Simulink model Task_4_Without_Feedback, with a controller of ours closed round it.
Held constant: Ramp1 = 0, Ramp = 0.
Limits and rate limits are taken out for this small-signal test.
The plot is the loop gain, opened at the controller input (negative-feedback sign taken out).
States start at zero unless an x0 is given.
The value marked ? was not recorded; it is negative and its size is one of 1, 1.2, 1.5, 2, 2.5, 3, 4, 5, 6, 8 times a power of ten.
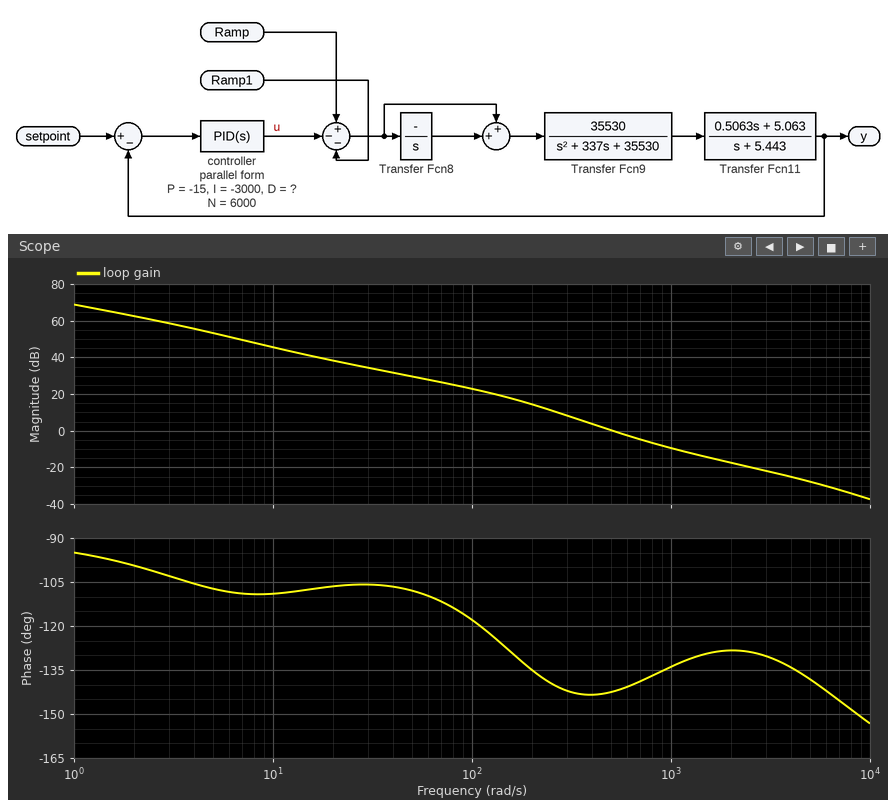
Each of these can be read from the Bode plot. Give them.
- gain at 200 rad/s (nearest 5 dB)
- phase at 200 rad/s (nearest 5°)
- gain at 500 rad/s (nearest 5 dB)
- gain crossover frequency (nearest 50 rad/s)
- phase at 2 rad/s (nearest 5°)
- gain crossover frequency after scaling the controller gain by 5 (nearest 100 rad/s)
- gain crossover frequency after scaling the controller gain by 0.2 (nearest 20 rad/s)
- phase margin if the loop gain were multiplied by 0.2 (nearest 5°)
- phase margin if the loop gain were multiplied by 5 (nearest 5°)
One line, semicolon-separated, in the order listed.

15 dB; -135°; 0 dB; 500 rad/s; -100°; 1500 rad/s; 200 rad/s; 45°; 50°
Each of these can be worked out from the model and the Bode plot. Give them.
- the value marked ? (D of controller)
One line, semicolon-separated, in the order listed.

-0.012
